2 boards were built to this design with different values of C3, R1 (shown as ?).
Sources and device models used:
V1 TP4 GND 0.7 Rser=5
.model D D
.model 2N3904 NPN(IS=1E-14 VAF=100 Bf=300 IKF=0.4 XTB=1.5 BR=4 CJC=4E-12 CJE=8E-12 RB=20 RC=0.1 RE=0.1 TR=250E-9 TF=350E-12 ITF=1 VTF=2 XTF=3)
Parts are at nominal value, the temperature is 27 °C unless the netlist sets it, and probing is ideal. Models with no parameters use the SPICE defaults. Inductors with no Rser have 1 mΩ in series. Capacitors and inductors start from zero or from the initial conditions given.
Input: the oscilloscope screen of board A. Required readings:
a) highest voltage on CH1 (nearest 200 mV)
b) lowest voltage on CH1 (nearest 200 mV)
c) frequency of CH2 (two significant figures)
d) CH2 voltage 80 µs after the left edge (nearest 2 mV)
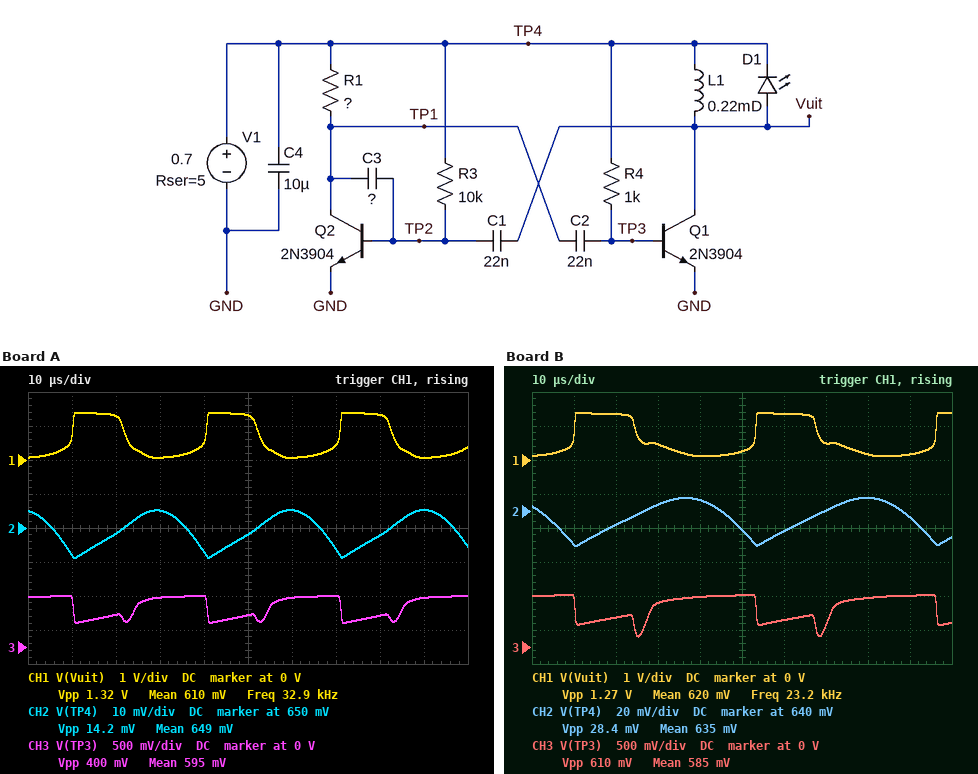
1.4 V
0 V
33 kHz
648 mV
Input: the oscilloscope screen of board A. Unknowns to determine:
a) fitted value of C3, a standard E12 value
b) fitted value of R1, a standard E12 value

47 nF
100 Ω
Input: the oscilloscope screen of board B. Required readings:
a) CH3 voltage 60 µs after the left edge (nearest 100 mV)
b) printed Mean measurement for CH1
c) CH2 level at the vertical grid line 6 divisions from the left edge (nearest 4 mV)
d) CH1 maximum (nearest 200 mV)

400 mV
620 mV
628 mV
1.4 V
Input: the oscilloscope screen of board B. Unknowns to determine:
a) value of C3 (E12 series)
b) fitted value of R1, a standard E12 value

47 nF
270 Ω
